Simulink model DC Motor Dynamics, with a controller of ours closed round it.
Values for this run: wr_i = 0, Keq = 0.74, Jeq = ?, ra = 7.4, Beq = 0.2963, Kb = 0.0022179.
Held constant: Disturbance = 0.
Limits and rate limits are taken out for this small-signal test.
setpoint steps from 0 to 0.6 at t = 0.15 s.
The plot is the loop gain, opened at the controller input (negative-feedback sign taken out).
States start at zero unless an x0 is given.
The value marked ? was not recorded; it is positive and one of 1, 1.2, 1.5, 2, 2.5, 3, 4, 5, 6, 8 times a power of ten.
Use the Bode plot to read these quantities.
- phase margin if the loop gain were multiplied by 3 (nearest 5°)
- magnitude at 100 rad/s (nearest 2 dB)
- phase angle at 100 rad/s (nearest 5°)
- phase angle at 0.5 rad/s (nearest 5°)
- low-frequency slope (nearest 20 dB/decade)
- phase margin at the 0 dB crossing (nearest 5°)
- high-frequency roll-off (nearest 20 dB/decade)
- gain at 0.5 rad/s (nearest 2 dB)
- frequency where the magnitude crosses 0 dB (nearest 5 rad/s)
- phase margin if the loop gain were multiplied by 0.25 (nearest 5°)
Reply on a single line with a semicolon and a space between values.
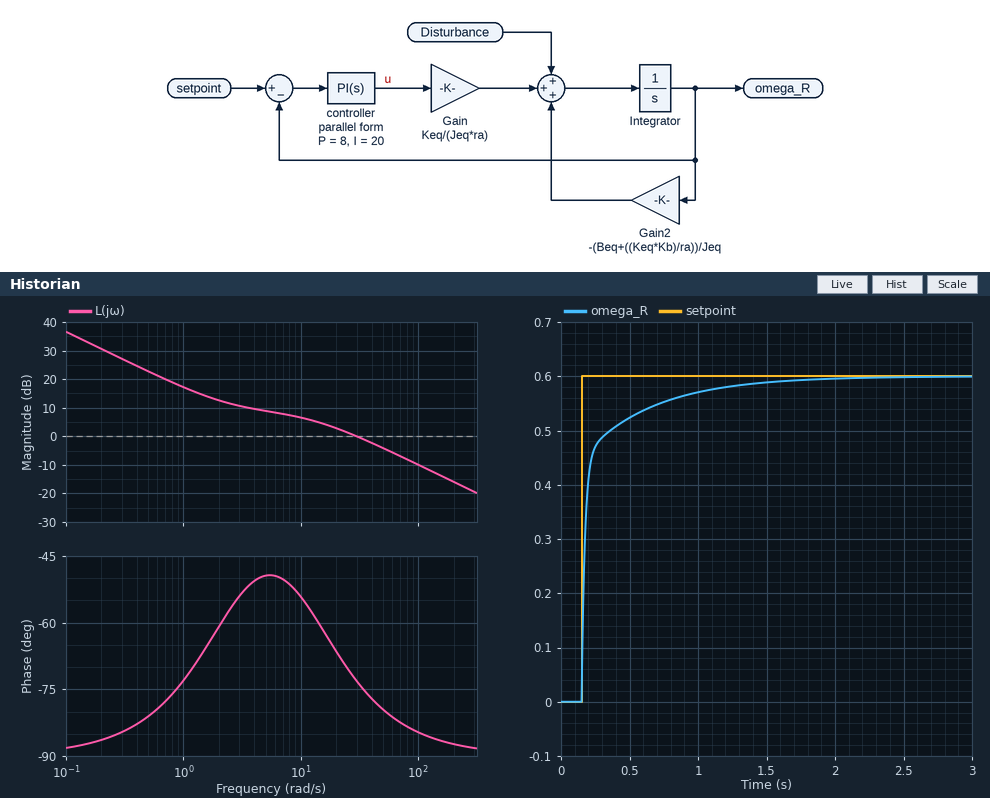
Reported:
95°; -10 dB; -85°; -80°; -20 dB/decade; 105°; -20 dB/decade; 22 dB; 30 rad/s; 120°
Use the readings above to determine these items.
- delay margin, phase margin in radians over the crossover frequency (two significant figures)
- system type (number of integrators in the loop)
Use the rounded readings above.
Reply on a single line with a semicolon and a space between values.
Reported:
0.061 s; 1
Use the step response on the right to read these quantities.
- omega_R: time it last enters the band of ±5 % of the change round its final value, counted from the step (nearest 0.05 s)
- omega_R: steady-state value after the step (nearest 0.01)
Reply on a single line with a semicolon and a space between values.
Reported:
0.85 s; 0.60
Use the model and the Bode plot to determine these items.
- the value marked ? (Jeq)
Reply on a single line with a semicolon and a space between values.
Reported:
0.025
